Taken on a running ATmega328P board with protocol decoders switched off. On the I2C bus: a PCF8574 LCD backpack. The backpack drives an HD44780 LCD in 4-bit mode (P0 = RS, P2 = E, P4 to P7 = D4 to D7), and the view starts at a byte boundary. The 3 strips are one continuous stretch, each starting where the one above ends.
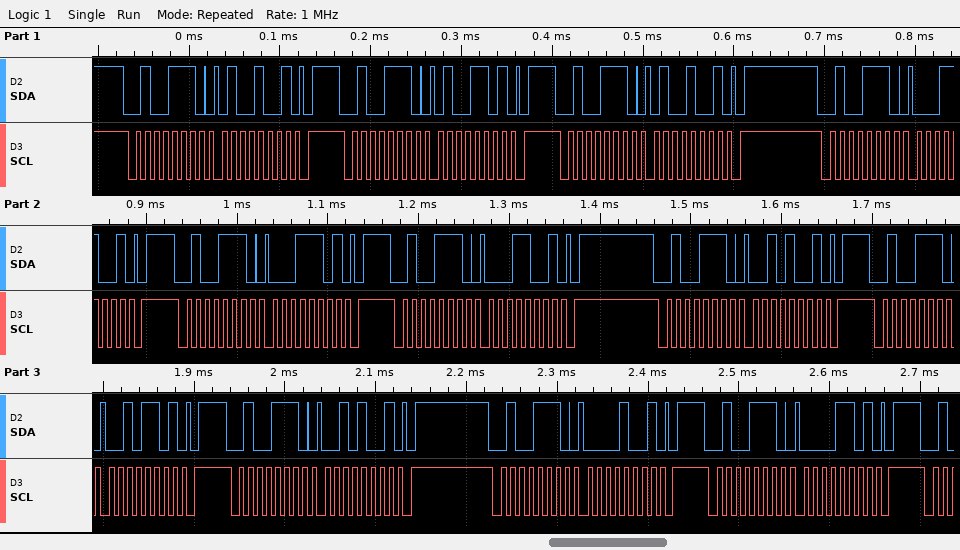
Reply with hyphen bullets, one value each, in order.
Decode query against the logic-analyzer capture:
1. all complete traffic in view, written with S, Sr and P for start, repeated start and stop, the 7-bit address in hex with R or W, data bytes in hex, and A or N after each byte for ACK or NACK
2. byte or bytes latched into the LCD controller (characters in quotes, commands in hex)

- S 27W A 49 A P S 27W A 4D A P S 27W A 49 A P S 27W A 19 A P S 27W A 1D A P S 27W A 19 A P S 27W A 29 A P S 27W A 2D A P S 27W A 29 A P S 27W A 09 A P S 27W A 0D A P
- 'A'
